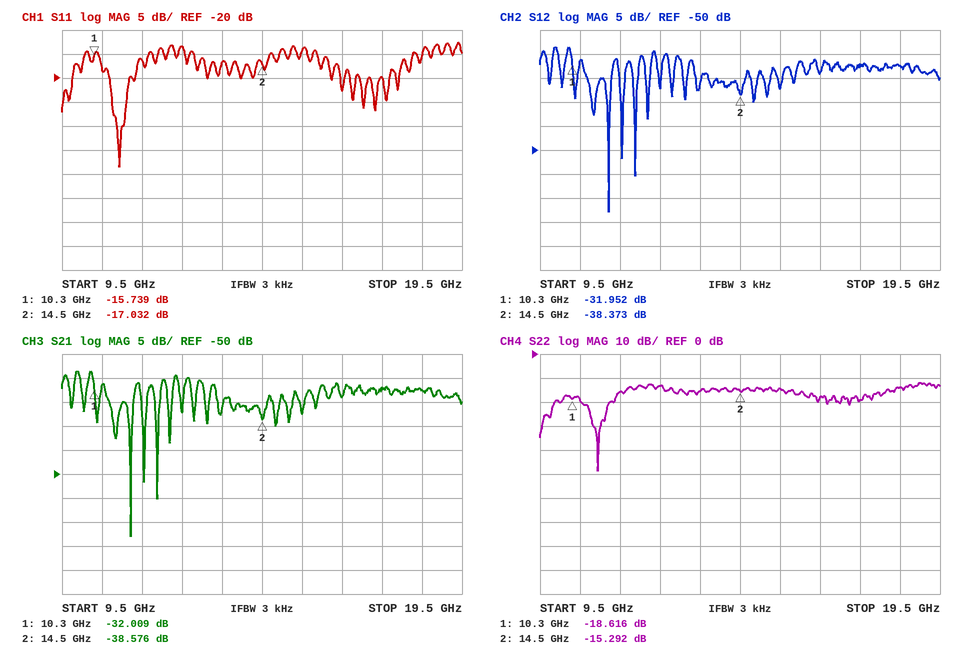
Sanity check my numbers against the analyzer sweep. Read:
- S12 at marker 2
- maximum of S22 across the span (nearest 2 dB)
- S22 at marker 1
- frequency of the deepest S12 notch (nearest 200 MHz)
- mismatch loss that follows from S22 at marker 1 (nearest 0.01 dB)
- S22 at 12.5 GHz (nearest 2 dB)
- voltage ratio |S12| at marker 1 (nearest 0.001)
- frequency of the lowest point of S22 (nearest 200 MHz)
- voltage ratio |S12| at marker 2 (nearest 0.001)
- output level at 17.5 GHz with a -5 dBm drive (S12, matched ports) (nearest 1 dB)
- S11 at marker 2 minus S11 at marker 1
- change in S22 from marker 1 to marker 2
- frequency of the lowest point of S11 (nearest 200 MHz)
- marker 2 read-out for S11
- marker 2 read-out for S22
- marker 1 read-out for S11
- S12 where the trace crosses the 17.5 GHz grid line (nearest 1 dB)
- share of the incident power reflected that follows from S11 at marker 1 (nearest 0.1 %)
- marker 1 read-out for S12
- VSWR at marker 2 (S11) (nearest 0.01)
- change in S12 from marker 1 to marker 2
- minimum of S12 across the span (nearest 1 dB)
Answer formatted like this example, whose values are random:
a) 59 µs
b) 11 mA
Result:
a) -38.373 dB
b) -12 dB
c) -18.616 dB
d) 11.2 GHz
e) 0.06 dB
f) -14 dB
g) 0.025
h) 11.0 GHz
i) 0.012
j) -37 dBm
k) -1.293 dB
l) 3.324 dB
m) 11.0 GHz
n) -17.032 dB
o) -15.292 dB
p) -15.739 dB
q) -32 dB
r) 2.7 %
s) -31.952 dB
t) 1.33
u) -6.421 dB
v) -63 dB
